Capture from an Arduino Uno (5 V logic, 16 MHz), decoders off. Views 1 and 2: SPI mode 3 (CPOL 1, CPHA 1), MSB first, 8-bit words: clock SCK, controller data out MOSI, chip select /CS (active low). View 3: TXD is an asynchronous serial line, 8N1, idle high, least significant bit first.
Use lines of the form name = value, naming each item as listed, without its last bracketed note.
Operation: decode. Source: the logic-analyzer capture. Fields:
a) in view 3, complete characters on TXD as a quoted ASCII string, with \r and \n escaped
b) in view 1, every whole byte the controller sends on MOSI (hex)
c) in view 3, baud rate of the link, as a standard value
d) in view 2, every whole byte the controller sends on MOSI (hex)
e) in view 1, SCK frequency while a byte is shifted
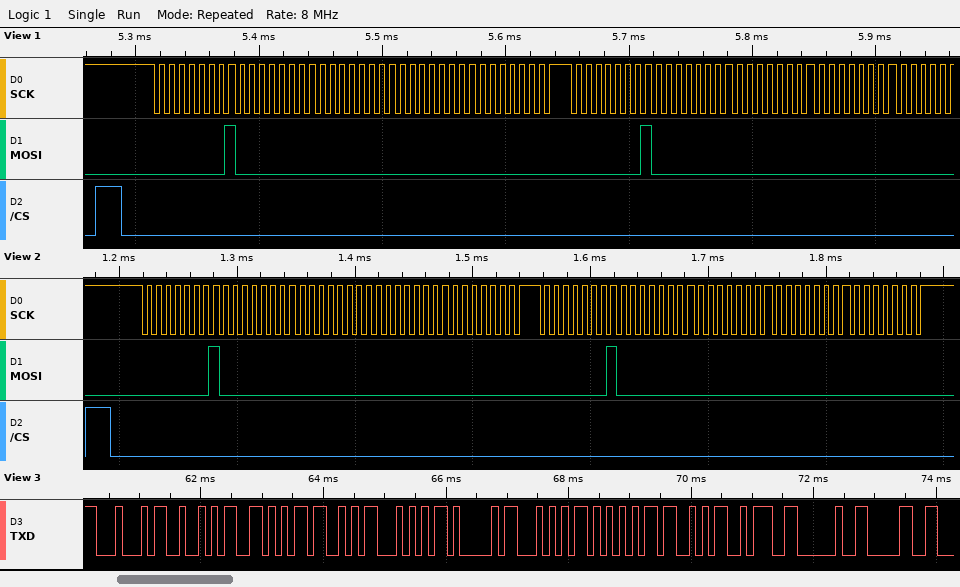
in view 3, complete characters on TXD as a quoted ASCII string, with \r and \n escaped = "DRVSTATUS: 0"
in view 1, every whole byte the controller sends on MOSI = 01 00 00 00 00 01 00 00 00
in view 3, baud rate of the link, as a standard value = 9600 baud
in view 2, every whole byte the controller sends on MOSI = 01 00 00 00 00 01 00 00 00 00
in view 1, SCK frequency while a byte is shifted = 125 kHz
